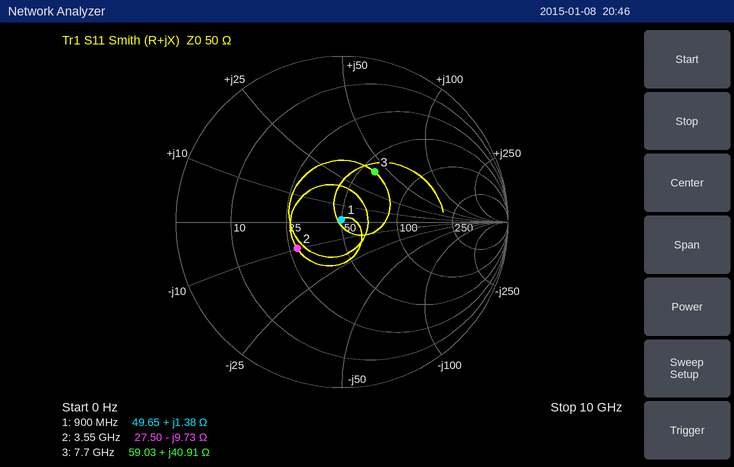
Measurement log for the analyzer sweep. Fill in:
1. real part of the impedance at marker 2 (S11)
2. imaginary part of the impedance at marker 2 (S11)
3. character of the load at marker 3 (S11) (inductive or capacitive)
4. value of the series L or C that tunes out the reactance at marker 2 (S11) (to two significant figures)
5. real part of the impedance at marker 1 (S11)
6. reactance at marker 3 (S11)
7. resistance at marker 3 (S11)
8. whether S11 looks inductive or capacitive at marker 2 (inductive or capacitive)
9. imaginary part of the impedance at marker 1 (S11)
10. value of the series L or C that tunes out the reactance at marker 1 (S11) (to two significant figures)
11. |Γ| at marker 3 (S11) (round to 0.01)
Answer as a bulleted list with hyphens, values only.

- 27.50 Ω
- -9.73 Ω
- inductive
- 440 pH
- 49.65 Ω
- +40.91 Ω
- 59.03 Ω
- capacitive
- +1.38 Ω
- 130 pF
- 0.36
